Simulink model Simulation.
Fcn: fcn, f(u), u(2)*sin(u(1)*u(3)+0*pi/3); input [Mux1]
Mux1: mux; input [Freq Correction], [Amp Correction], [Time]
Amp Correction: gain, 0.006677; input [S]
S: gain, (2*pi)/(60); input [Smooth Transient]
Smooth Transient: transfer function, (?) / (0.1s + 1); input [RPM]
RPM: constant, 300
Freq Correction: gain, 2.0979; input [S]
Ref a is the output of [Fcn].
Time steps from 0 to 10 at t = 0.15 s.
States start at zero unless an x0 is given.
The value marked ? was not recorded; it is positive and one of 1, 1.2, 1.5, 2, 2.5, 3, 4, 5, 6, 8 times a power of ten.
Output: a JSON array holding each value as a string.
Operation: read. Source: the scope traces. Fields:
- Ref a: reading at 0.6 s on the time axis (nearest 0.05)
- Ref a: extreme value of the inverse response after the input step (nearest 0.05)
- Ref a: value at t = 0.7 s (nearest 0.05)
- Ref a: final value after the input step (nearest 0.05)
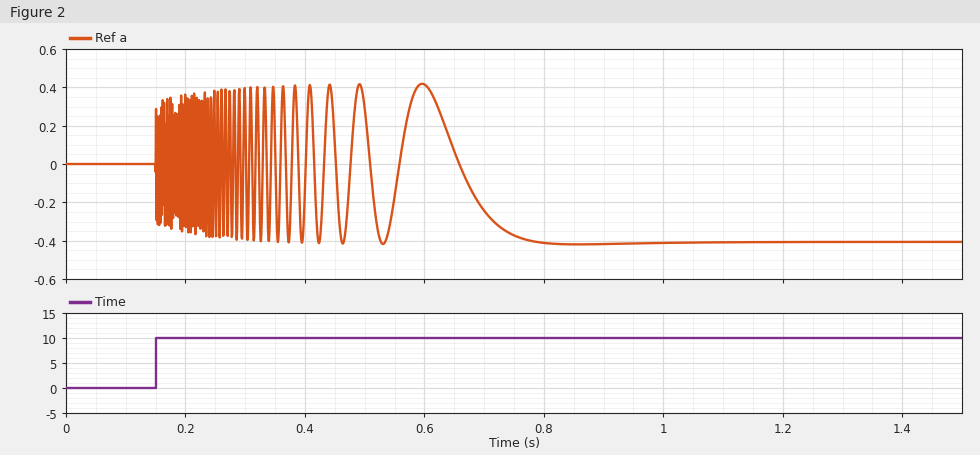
["0.40", "0.40", "-0.25", "-0.40"]
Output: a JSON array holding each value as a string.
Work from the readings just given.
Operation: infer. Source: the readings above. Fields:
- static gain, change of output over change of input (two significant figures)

["-0.040"]
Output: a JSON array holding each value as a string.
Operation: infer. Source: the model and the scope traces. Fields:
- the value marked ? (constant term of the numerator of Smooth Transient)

["2"]
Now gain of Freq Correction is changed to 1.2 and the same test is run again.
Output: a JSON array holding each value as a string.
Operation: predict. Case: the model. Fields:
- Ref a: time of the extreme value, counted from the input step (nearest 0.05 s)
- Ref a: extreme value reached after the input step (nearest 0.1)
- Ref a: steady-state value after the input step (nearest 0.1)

["0.45 s", "-0.4", "0.0"]
